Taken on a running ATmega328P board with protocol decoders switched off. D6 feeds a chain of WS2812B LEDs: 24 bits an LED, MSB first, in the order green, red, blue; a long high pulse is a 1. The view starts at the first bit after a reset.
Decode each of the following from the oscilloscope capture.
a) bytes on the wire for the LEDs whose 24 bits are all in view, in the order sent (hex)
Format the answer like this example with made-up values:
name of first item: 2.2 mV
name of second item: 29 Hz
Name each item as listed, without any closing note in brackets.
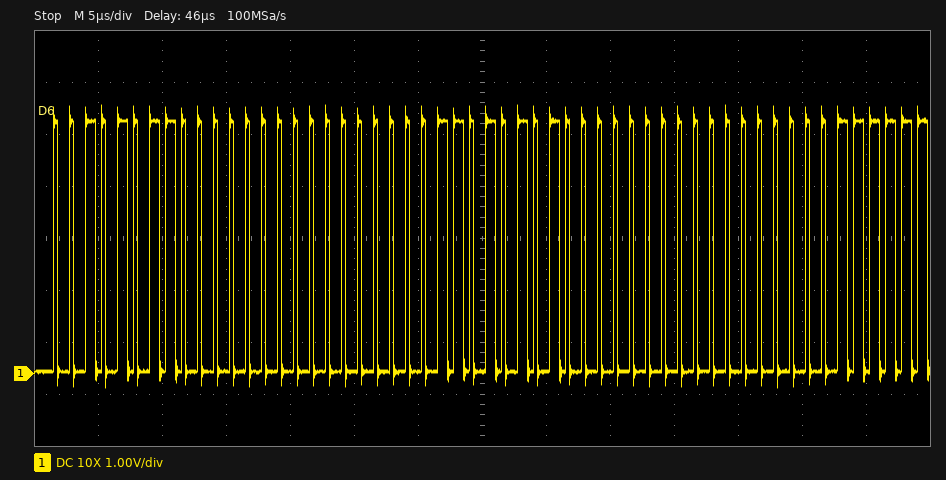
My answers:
bytes on the wire for the LEDs whose 24 bits are all in view, in the order sent: 2B 00 00 D5 00 00
